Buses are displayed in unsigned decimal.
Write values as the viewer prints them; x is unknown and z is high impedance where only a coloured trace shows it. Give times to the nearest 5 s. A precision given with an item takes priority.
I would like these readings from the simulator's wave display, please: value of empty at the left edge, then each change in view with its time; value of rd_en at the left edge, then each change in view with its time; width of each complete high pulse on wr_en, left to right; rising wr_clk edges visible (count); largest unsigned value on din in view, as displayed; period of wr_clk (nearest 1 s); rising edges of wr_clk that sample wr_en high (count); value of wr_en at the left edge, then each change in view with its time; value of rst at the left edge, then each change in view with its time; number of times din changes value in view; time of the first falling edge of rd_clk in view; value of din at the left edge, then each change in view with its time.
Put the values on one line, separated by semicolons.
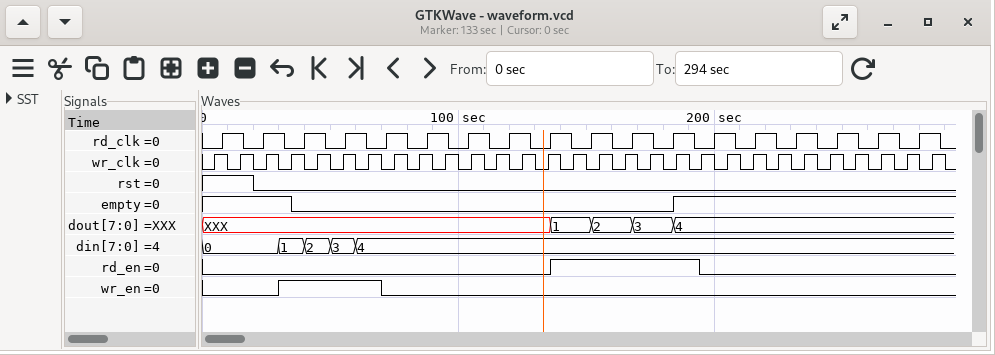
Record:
1, 0 at 35 s, 1 at 185 s; 0, 1 at 135 s, 0 at 195 s; 40 s; 29; 4; 10 s; 4; 0, 1 at 30 s, 0 at 70 s; 1, 0 at 20 s; 4; 15 s; 0, 1 at 30 s, 2 at 40 s, 3 at 50 s, 4 at 60 s
